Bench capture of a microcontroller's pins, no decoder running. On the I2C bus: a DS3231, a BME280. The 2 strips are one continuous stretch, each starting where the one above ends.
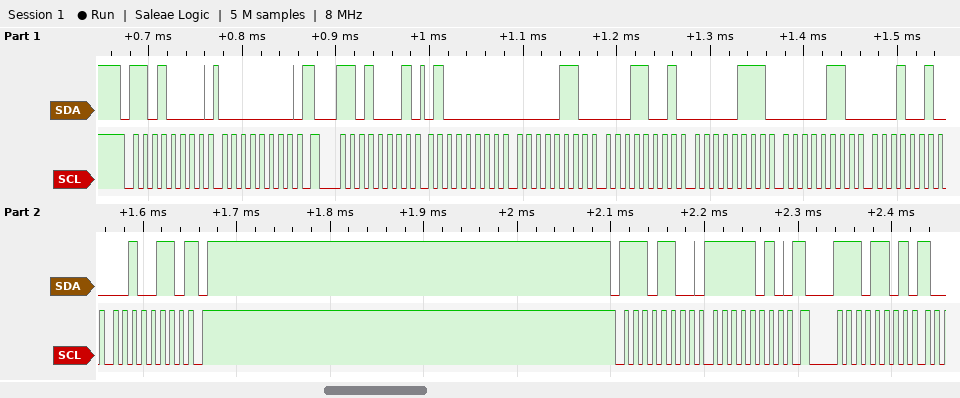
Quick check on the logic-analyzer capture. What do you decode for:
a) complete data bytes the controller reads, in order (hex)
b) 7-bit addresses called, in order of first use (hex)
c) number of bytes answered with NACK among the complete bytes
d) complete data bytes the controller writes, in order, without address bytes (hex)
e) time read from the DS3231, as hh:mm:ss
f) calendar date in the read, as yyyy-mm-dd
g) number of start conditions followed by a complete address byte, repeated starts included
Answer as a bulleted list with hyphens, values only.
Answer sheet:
- 40 06 19 07 06 12 26
- 0x68 0x76
- 1
- 00 FA
- 19:06:40
- 2026-12-06
- 4
